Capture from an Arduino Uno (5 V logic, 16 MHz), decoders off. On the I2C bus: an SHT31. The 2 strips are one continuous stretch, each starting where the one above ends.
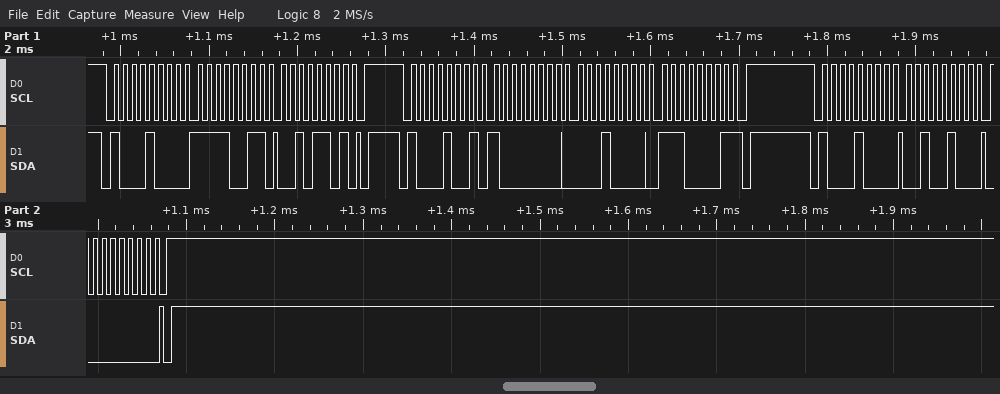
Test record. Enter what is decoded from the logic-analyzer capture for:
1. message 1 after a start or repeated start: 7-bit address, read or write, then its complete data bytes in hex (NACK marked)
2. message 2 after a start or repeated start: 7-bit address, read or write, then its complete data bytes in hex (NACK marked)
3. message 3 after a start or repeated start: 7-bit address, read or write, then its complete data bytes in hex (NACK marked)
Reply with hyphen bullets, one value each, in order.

- 0x44 write: F3 2D
- 0x44 read: 80 10 E1 NACK
- 0x44 write: 24 00
